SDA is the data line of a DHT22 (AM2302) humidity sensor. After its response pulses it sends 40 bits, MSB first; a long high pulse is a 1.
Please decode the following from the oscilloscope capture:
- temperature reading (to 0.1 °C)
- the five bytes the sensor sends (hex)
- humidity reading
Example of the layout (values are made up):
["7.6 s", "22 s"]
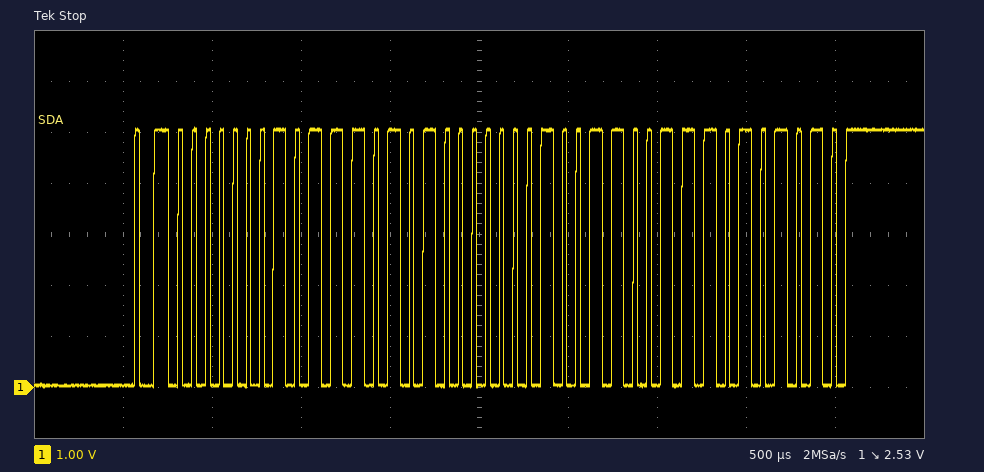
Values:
["30.7 °C", "01 75 01 33 AA", "37.3 %"]
